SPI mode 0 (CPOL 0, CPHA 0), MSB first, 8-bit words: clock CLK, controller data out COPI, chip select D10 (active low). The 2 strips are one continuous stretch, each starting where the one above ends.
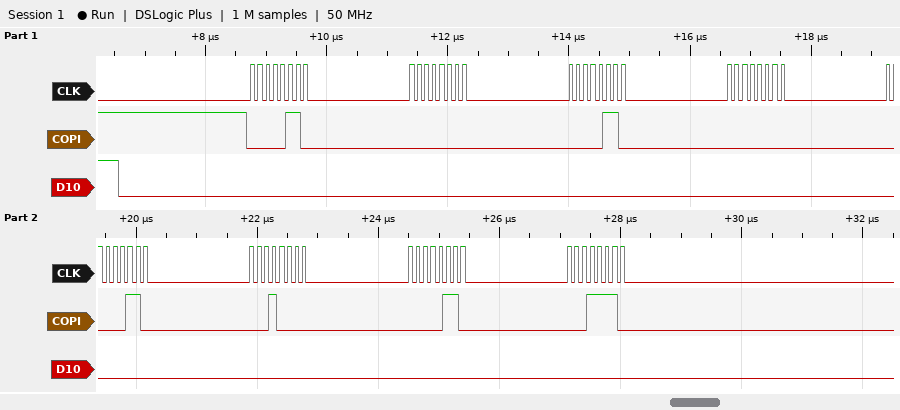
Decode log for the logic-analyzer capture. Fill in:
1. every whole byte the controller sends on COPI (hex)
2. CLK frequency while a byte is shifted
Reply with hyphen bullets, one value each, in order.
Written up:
- 06 00 06 00 06 10 06 1E
- 8 MHz
